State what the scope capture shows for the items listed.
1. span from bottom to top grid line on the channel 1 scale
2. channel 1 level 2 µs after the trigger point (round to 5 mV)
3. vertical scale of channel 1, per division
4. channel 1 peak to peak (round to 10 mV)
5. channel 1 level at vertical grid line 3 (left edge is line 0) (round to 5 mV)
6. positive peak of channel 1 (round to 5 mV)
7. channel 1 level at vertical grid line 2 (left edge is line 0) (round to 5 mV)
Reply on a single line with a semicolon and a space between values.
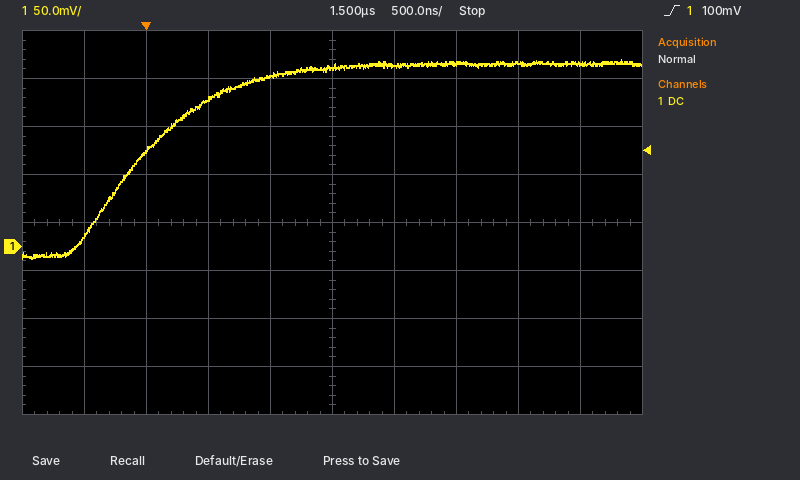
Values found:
400 mV; 190 mV; 50 mV; 210 mV; 155 mV; 195 mV; 100 mV
